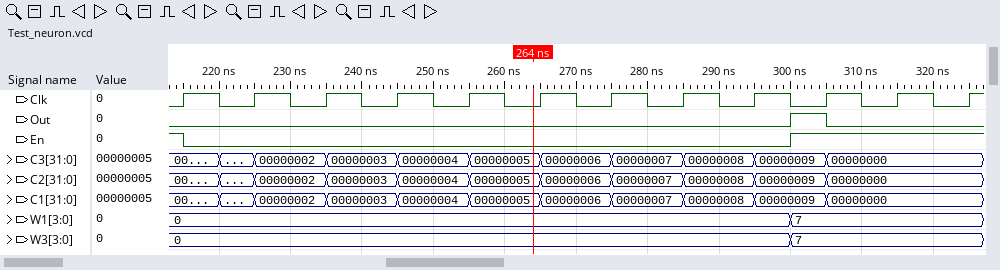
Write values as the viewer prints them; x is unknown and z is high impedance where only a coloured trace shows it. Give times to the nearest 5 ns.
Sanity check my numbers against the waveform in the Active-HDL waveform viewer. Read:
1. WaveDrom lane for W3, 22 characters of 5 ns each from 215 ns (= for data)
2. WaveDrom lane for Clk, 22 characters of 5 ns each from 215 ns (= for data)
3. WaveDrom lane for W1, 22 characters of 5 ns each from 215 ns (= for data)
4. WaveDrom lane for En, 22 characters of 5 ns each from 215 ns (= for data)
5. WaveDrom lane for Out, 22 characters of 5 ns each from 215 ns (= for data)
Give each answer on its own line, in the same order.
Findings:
{name: 'W3', wave: '=................=....', data: '0 7'}
{name: 'Clk', wave: '1010101010101010101010'}
{name: 'W1', wave: '=................=....', data: '0 7'}
{name: 'En', wave: '0................1....'}
{name: 'Out', wave: '0................10...'}
